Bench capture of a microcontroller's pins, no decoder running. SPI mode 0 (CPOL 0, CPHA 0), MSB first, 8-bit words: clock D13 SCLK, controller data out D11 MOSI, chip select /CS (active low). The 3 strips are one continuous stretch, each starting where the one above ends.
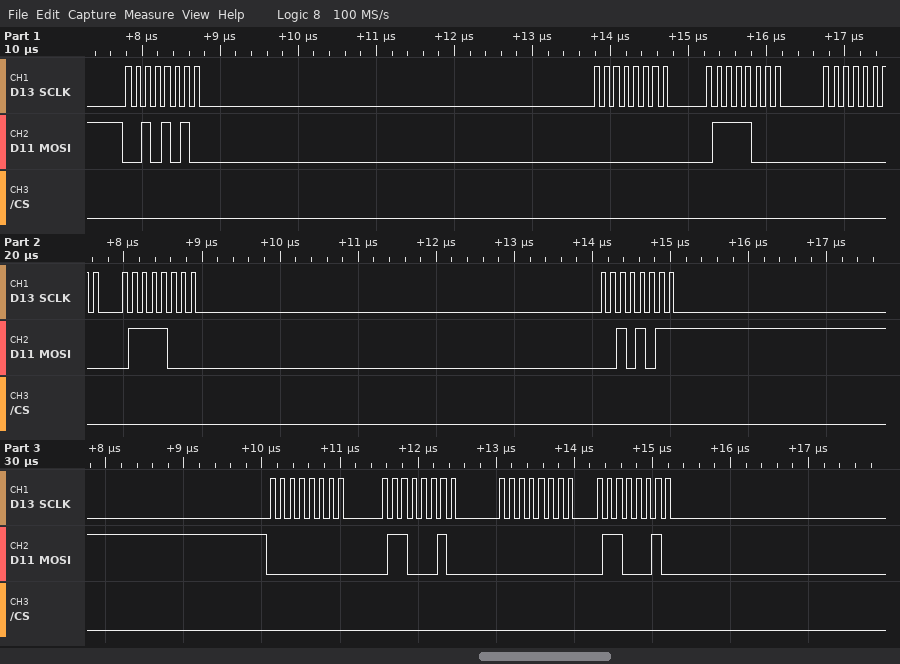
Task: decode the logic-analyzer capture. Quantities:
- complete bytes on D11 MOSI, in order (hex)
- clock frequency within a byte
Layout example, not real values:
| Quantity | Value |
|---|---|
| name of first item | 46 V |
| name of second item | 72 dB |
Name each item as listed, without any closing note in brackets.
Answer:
| Quantity | Value |
|---|---|
| complete bytes on D11 MOSI, in order | 2A 00 78 00 78 2B 00 62 00 62 |
| clock frequency within a byte | 8 MHz |
